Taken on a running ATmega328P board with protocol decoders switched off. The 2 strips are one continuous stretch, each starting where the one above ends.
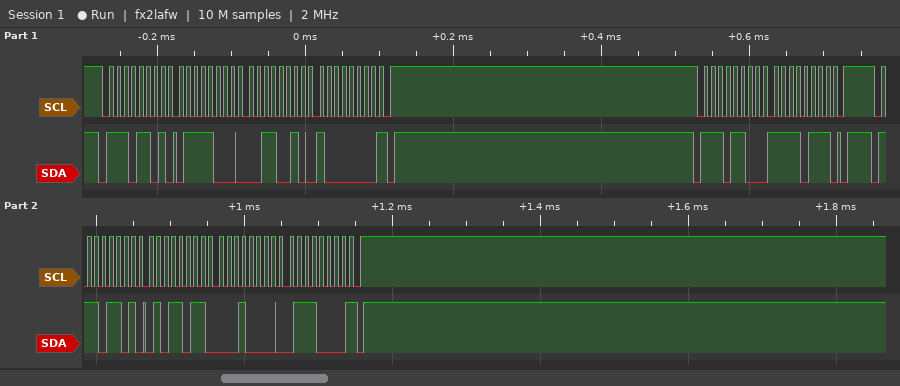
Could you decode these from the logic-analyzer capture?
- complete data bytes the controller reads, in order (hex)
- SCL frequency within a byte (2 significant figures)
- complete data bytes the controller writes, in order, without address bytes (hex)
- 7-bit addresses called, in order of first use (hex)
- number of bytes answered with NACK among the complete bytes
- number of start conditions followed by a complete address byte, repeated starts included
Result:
78 32 80 5B 10 70
100 kHz
F7
0x76
2
3
